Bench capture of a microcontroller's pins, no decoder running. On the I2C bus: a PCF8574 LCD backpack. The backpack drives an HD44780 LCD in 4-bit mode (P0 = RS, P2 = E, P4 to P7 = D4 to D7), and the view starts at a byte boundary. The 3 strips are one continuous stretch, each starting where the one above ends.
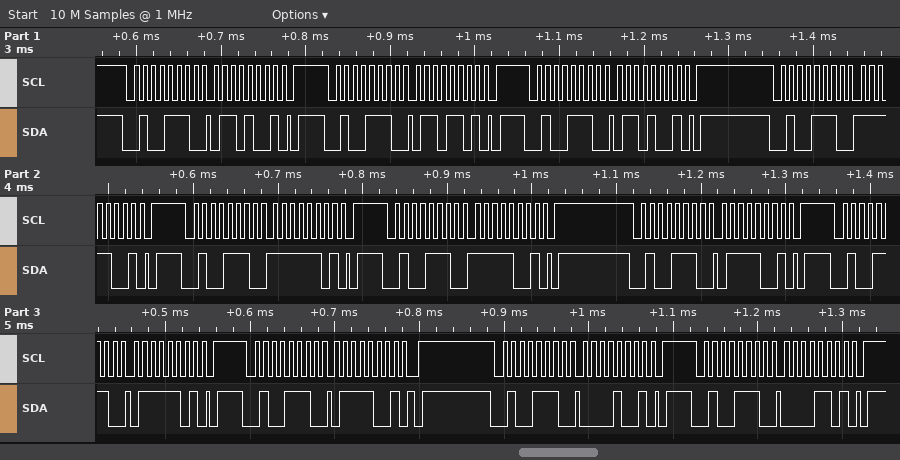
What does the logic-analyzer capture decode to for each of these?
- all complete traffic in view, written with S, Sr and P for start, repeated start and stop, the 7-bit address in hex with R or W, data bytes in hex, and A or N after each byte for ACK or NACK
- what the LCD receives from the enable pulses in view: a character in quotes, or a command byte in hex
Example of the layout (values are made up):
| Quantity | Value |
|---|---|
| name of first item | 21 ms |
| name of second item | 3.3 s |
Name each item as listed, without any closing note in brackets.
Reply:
| Quantity | Value |
|---|---|
| all complete traffic in view, written with S, Sr and P for start, repeated start and stop, the 7-bit address in hex with R or W, data bytes in hex, and A or N after each byte for ACK or NACK | S 27W A 69 A P S 27W A 6D A P S 27W A 69 A P S 27W A F9 A P S 27W A FD A P S 27W A F9 A P S 27W A 79 A P S 27W A 7D A P S 27W A 79 A P S 27W A 09 A P S 27W A 0D A P |
| what the LCD receives from the enable pulses in view: a character in quotes, or a command byte in hex | 'o' |
